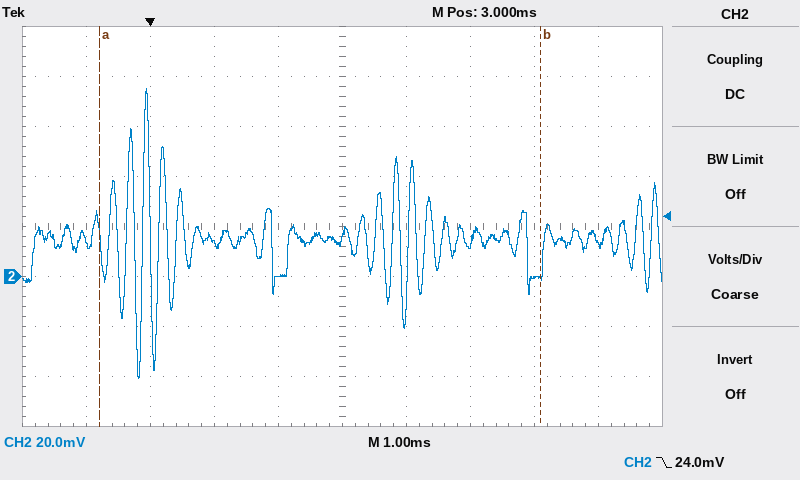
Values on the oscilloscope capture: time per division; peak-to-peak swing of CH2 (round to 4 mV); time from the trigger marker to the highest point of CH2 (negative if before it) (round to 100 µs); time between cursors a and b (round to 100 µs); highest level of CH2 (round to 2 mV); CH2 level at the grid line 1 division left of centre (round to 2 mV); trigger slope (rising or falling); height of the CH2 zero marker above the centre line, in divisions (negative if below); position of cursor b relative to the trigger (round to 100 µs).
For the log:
1 ms
116 mV
-100 µs
6.9 ms
76 mV
0 mV
falling
-1.0 div
+6.1 ms
